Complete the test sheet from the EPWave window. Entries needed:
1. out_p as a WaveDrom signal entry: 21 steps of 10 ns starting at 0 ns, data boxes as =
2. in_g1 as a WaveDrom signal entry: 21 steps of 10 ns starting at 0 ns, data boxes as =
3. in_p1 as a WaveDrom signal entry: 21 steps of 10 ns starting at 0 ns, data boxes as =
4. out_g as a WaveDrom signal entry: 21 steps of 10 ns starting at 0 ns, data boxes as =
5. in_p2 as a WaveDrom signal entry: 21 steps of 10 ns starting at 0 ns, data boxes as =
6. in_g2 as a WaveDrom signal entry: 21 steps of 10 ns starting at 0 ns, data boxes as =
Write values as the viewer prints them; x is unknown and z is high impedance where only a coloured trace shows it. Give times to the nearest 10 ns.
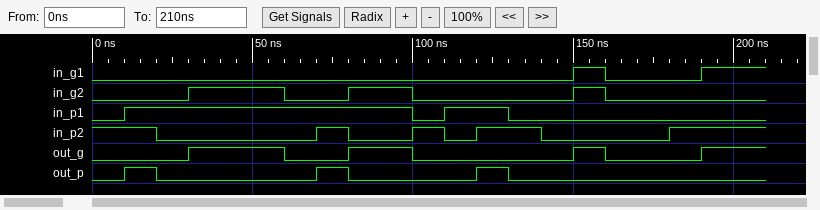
{name: 'out_p', wave: '010....10...10.......'}
{name: 'in_g1', wave: '0..............10..1.'}
{name: 'in_p1', wave: '01........01.0.......'}
{name: 'out_g', wave: '0..1..0.1.0....10..1.'}
{name: 'in_p2', wave: '1.0....10.101.0...1..'}
{name: 'in_g2', wave: '0..1..0.1.0....10....'}
